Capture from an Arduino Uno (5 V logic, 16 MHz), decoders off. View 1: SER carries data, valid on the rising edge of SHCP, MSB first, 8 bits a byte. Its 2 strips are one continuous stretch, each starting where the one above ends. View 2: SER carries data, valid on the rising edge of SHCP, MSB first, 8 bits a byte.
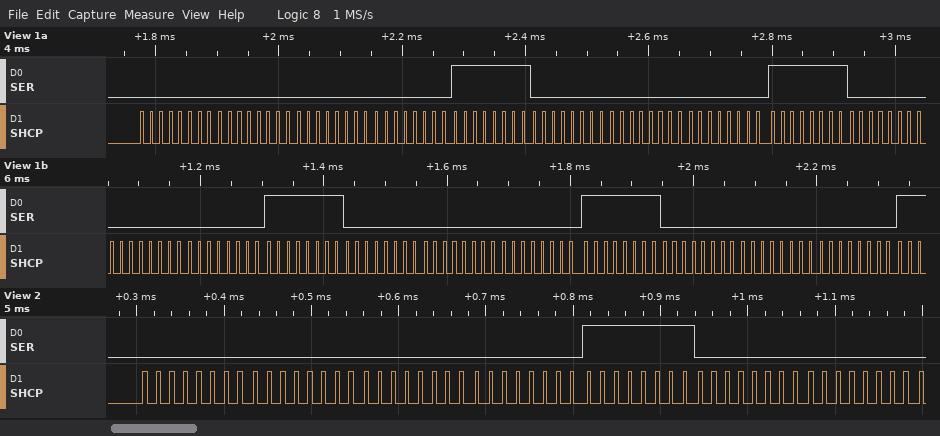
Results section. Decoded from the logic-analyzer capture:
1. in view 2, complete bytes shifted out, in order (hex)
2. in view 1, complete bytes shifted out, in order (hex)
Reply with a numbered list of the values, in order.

1. 00 00 00 00 FF 00 00
2. 0x00 0x00 0x00 0x00 0xFF 0x00 0x00 0x00 0xFF 0x00 0x00 0x00 0xFF 0x00 0x00 0x00 0xFF 0x00 0x00 0x00
